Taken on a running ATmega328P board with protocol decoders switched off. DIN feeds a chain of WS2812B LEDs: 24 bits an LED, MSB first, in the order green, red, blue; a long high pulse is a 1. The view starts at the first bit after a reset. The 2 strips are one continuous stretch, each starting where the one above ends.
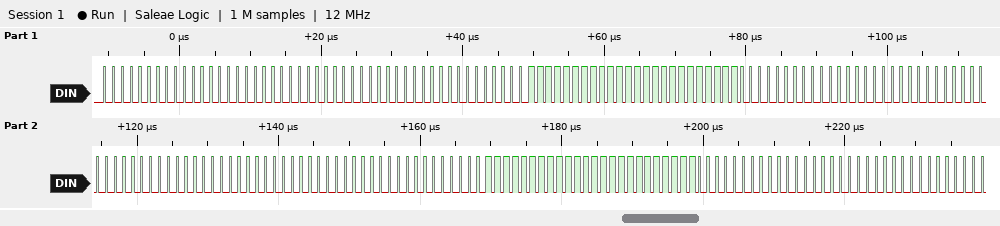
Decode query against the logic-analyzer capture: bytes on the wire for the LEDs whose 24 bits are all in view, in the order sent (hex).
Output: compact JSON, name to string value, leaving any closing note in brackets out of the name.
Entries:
{"bytes on the wire for the LEDs whose 24 bits are all in view, in the order sent": "00 00 00 00 00 00 FF FF FF 00 00 00 00 00 00 00 00 00 FF FF FF 00 00 00"}
